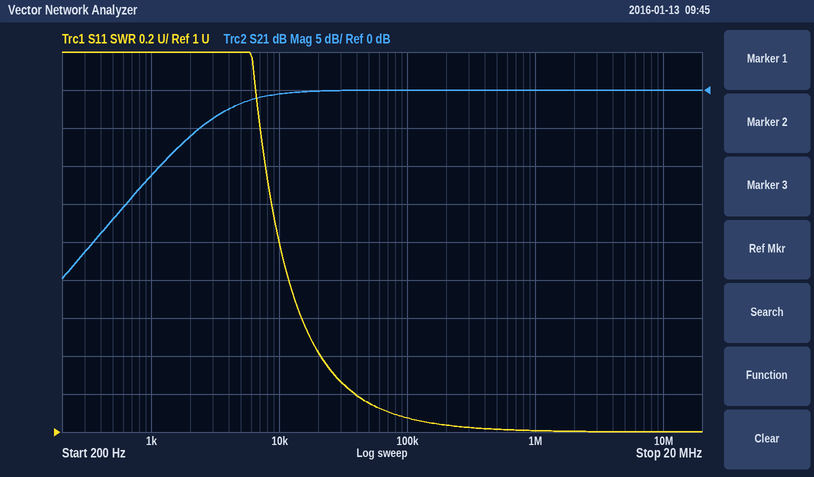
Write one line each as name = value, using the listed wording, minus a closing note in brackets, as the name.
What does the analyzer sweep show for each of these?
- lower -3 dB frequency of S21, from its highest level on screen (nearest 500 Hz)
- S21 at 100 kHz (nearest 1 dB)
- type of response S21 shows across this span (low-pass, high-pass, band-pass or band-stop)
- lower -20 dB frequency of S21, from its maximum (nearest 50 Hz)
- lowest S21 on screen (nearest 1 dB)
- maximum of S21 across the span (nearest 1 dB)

lower -3 dB frequency of S21, from its highest level on screen = 3.5 kHz
S21 at 100 kHz = 0 dB
type of response S21 shows across this span = high-pass
lower -20 dB frequency of S21, from its maximum = 350 Hz
lowest S21 on screen = -25 dB
maximum of S21 across the span = 0 dB
